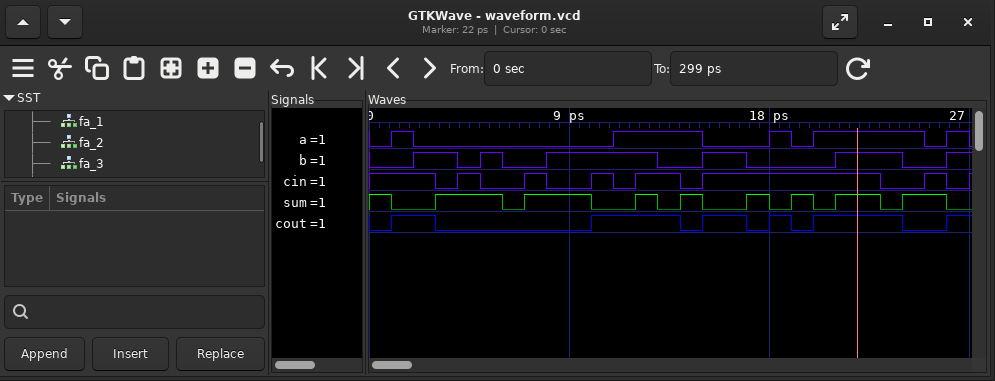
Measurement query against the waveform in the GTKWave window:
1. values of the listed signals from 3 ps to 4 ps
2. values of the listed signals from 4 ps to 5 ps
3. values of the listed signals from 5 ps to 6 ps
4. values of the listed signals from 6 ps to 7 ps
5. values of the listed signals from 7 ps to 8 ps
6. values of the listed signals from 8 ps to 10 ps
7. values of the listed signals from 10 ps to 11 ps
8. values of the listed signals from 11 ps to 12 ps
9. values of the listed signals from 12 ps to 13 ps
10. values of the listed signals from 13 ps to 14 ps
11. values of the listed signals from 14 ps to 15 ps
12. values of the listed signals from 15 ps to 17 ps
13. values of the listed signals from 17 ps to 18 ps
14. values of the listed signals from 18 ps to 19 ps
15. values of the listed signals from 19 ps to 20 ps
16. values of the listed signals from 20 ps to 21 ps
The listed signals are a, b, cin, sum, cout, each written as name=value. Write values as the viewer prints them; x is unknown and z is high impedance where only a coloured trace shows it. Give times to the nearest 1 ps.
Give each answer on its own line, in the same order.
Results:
a=0, b=1, cin=0, sum=1, cout=0
a=0, b=0, cin=1, sum=1, cout=0
a=0, b=1, cin=0, sum=1, cout=0
a=0, b=0, cin=0, sum=0, cout=0
a=0, b=0, cin=1, sum=1, cout=0
a=0, b=1, cin=0, sum=1, cout=0
a=0, b=1, cin=1, sum=0, cout=1
a=1, b=1, cin=0, sum=0, cout=1
a=1, b=1, cin=1, sum=1, cout=1
a=1, b=0, cin=1, sum=0, cout=1
a=1, b=0, cin=0, sum=1, cout=0
a=0, b=1, cin=1, sum=0, cout=1
a=0, b=0, cin=1, sum=1, cout=0
a=1, b=0, cin=1, sum=0, cout=1
a=0, b=0, cin=1, sum=1, cout=0
a=1, b=0, cin=1, sum=0, cout=1
